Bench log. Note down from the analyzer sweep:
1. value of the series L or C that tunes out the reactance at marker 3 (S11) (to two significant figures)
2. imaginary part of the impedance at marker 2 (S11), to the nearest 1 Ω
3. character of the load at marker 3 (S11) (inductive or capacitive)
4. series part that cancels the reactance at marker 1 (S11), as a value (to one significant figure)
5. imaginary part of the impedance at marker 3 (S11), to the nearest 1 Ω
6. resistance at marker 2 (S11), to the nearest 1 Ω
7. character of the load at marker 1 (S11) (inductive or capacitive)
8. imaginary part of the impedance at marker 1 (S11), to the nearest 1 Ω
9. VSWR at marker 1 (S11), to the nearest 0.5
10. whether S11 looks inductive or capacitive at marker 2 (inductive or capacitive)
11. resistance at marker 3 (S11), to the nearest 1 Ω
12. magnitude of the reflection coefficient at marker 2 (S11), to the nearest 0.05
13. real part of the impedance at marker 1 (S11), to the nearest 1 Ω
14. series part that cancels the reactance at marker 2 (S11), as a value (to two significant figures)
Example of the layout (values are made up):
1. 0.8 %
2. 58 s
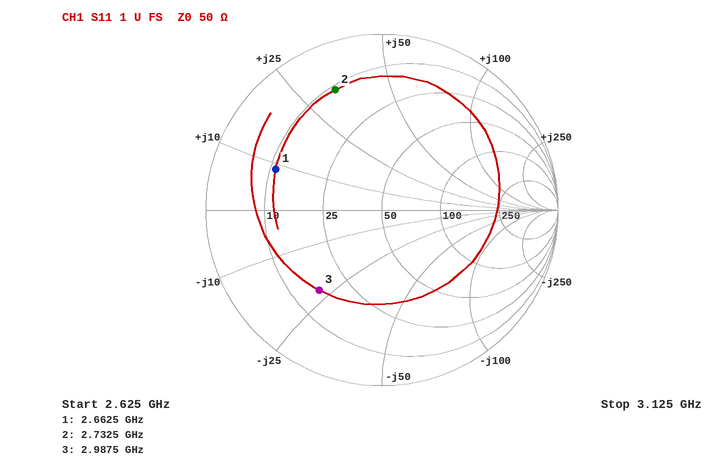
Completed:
1. 1.2 nH
2. +33 Ω
3. capacitive
4. 7 pF
5. -22 Ω
6. 11 Ω
7. inductive
8. +9 Ω
9. 4.5
10. inductive
11. 16 Ω
12. 0.75
13. 11 Ω
14. 1.8 pF
